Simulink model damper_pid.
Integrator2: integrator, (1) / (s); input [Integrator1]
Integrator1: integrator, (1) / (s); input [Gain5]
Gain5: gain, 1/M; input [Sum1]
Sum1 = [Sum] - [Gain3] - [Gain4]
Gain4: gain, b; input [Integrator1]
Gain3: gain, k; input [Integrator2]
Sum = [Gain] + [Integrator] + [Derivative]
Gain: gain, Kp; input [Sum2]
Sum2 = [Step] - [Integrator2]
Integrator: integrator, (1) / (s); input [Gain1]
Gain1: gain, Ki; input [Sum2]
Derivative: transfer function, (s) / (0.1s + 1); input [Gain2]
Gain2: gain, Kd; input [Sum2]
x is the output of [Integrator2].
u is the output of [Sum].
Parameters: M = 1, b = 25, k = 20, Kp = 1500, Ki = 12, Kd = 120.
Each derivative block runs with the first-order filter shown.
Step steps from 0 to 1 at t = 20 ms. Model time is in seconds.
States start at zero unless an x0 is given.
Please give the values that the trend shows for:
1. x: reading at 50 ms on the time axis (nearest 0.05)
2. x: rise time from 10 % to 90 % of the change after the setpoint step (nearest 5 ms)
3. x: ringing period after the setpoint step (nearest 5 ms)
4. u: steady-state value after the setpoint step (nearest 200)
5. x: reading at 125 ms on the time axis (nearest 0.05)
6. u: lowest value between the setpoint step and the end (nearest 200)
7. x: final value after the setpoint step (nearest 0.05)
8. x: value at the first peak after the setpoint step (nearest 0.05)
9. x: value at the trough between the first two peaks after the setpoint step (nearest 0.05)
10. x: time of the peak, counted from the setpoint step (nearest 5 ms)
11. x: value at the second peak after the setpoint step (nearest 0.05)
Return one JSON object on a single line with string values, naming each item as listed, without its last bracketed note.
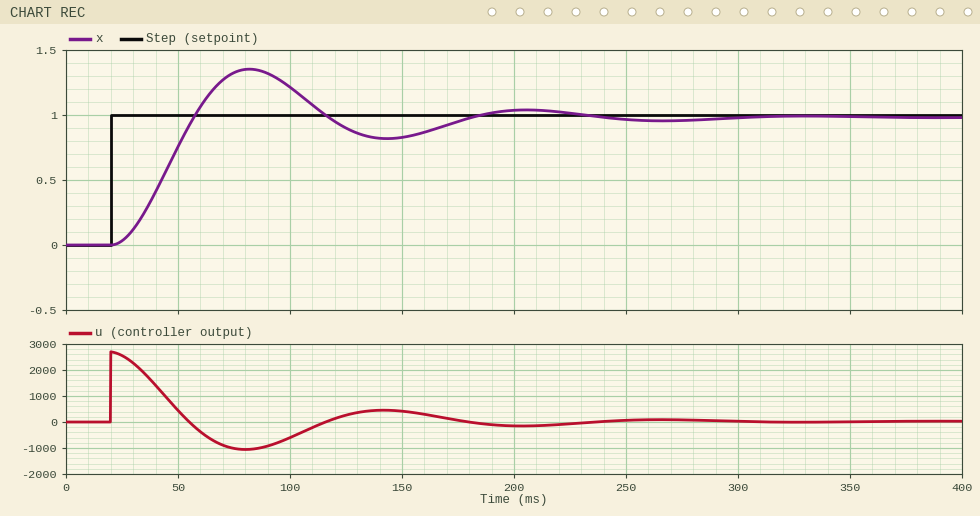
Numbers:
{"x: reading at 50 ms on the time axis": "0.75", "x: rise time from 10 % to 90 % of the change after the setpoint step": "25 ms", "x: ringing period after the setpoint step": "125 ms", "u: steady-state value after the setpoint step": "0", "x: reading at 125 ms on the time axis": "0.90", "u: lowest value between the setpoint step and the end": "-1000", "x: final value after the setpoint step": "1.00", "x: value at the first peak after the setpoint step": "1.35", "x: value at the trough between the first two peaks after the setpoint step": "0.80", "x: time of the peak, counted from the setpoint step": "60 ms", "x: value at the second peak after the setpoint step": "1.05"}
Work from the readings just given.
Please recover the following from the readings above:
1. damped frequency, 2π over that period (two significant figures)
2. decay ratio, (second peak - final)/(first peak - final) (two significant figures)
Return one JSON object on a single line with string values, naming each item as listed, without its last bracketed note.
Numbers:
{"damped frequency, 2π over that period": "0.050 rad/ms", "decay ratio, (second peak - final)/(first peak - final)": "0.14"}
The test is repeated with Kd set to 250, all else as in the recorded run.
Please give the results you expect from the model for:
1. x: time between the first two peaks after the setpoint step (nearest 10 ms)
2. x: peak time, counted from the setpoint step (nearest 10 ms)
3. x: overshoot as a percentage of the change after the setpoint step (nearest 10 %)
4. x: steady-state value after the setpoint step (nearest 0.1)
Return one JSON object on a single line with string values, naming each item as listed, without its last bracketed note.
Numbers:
{"x: time between the first two peaks after the setpoint step": "100 ms", "x: peak time, counted from the setpoint step": "50 ms", "x: overshoot as a percentage of the change after the setpoint step": "40 %", "x: steady-state value after the setpoint step": "1.0"}
